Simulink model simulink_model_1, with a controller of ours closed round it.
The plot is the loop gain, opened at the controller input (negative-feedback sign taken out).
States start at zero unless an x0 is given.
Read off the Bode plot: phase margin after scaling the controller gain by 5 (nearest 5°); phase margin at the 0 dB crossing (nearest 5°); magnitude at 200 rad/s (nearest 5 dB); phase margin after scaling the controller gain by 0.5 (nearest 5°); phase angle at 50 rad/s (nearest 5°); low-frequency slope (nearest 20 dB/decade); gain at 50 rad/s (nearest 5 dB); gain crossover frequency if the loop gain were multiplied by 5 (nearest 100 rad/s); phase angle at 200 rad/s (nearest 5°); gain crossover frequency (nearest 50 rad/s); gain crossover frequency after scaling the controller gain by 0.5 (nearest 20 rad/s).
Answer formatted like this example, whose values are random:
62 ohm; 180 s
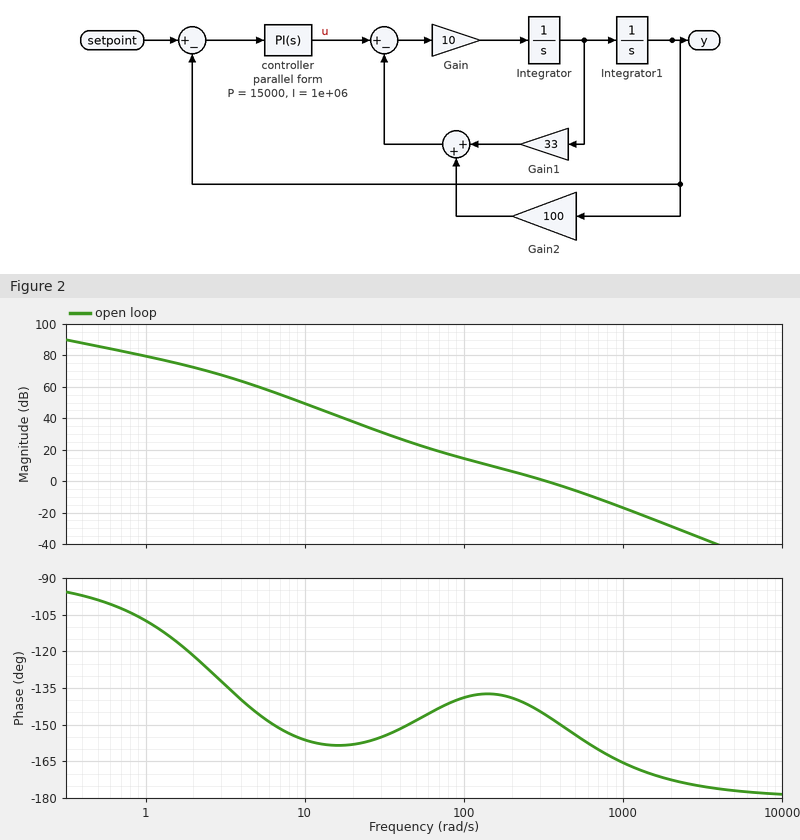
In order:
15°; 35°; 5 dB; 40°; -150°; -20 dB/decade; 25 dB; 800 rad/s; -140°; 350 rad/s; 200 rad/s
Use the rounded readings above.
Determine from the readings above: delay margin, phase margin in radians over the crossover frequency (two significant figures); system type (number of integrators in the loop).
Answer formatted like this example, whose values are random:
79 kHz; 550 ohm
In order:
0.0017 s; 1
